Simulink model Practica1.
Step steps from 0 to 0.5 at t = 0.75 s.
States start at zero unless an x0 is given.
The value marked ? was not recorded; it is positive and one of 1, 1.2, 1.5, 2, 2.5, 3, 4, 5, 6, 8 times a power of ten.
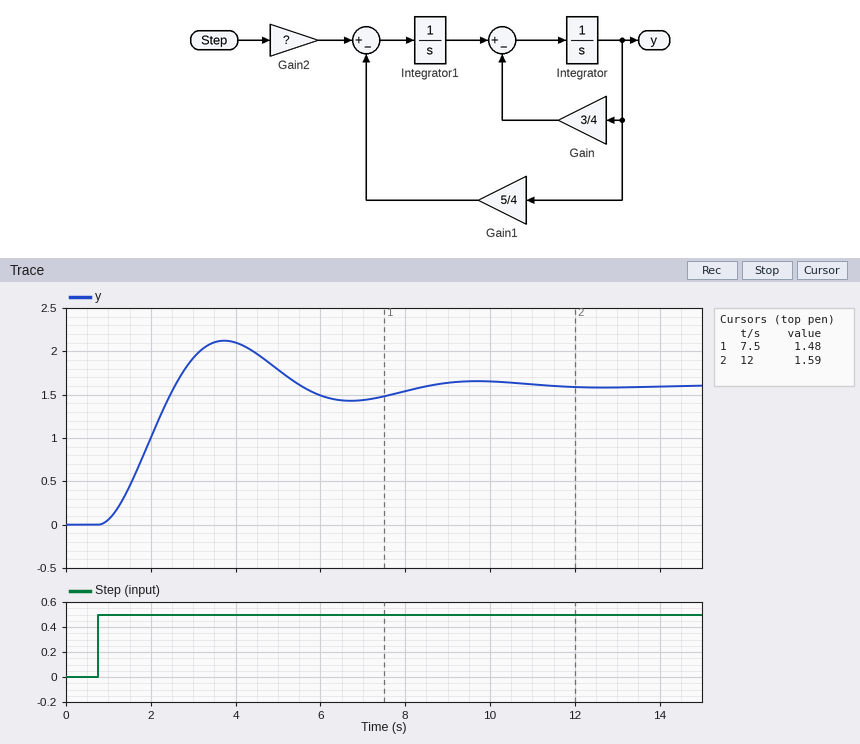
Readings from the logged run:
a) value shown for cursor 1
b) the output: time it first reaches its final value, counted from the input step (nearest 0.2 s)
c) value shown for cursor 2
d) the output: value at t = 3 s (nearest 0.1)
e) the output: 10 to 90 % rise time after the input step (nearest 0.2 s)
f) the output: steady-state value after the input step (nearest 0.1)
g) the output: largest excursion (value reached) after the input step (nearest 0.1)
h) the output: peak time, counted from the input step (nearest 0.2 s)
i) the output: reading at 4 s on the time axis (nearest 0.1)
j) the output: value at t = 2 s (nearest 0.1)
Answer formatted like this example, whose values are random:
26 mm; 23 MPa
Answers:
1.48; 1.8 s; 1.59; 1.9; 1.2 s; 1.6; 2.1; 3.0 s; 2.1; 1.0
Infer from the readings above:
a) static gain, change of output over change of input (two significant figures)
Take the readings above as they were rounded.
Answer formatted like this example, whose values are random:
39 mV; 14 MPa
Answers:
3.2
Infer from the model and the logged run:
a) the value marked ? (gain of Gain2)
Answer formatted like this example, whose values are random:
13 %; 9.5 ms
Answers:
4
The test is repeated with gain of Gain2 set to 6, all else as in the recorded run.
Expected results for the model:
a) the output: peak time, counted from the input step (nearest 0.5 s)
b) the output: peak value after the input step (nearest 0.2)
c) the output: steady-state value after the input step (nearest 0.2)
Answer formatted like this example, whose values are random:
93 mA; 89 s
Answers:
3.0 s; 3.2; 2.4
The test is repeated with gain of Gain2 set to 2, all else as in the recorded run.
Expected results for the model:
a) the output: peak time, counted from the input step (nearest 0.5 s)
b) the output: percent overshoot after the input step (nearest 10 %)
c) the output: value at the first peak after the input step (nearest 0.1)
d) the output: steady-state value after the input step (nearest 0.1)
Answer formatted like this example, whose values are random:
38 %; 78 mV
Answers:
3.0 s; 30 %; 1.1; 0.8
